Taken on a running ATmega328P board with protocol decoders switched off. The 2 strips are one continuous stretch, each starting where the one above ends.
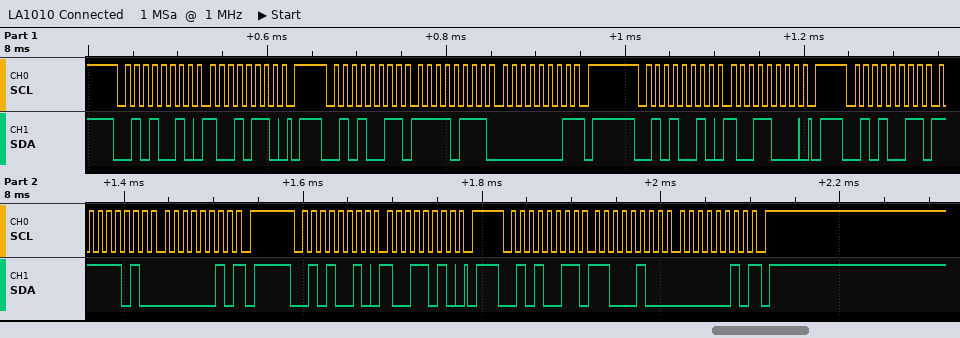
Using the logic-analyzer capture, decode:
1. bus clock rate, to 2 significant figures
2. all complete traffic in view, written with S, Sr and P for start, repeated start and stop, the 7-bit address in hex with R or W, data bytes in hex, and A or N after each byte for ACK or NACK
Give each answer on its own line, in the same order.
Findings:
100 kHz
S 29W A 96 A P S 29R A F7 A 01 N P S 29W A 98 A P S 29R A FA A 02 N P S 29W A 9A A P S 29R A C4 A 02 N P
